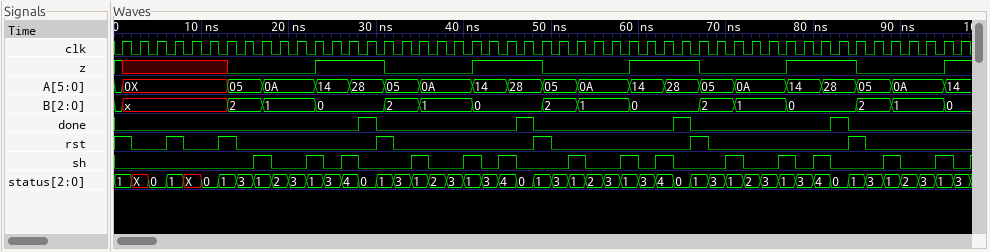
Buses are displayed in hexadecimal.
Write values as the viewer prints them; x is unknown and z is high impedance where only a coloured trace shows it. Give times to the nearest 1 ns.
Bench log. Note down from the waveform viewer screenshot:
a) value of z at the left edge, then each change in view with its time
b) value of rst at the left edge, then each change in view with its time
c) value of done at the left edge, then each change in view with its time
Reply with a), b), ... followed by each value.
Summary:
a) 1, x at 1 ns, 0 at 13 ns, 1 at 23 ns, 0 at 31 ns, 1 at 41 ns, 0 at 49 ns, 1 at 59 ns, 0 at 67 ns, 1 at 77 ns, 0 at 85 ns, 1 at 95 ns
b) 1, 0 at 2 ns, 1 at 6 ns, 0 at 8 ns, 1 at 12 ns, 0 at 14 ns, 1 at 30 ns, 0 at 32 ns, 1 at 48 ns, 0 at 50 ns, 1 at 66 ns, 0 at 68 ns, 1 at 84 ns, 0 at 86 ns
c) 0, 1 at 28 ns, 0 at 30 ns, 1 at 46 ns, 0 at 48 ns, 1 at 64 ns, 0 at 66 ns, 1 at 82 ns, 0 at 84 ns
